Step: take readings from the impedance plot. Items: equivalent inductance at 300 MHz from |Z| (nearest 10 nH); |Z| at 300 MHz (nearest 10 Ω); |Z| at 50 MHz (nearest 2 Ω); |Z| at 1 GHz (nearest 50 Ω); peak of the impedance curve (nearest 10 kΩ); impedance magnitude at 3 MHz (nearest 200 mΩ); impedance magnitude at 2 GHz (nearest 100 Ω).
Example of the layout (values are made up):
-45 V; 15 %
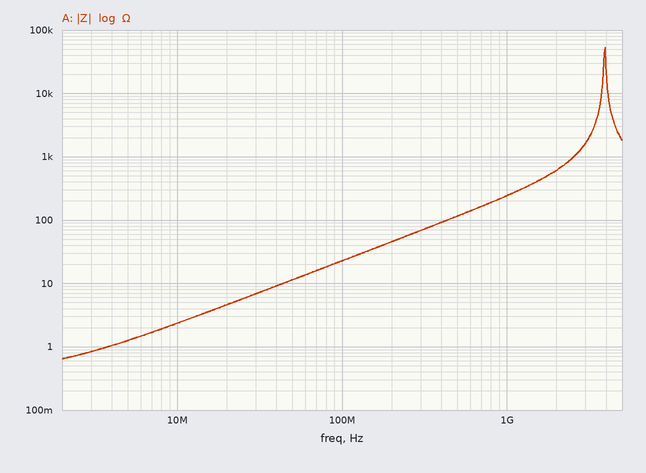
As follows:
40 nH; 70 Ω; 12 Ω; 250 Ω; 50 kΩ; 800 mΩ; 600 Ω
